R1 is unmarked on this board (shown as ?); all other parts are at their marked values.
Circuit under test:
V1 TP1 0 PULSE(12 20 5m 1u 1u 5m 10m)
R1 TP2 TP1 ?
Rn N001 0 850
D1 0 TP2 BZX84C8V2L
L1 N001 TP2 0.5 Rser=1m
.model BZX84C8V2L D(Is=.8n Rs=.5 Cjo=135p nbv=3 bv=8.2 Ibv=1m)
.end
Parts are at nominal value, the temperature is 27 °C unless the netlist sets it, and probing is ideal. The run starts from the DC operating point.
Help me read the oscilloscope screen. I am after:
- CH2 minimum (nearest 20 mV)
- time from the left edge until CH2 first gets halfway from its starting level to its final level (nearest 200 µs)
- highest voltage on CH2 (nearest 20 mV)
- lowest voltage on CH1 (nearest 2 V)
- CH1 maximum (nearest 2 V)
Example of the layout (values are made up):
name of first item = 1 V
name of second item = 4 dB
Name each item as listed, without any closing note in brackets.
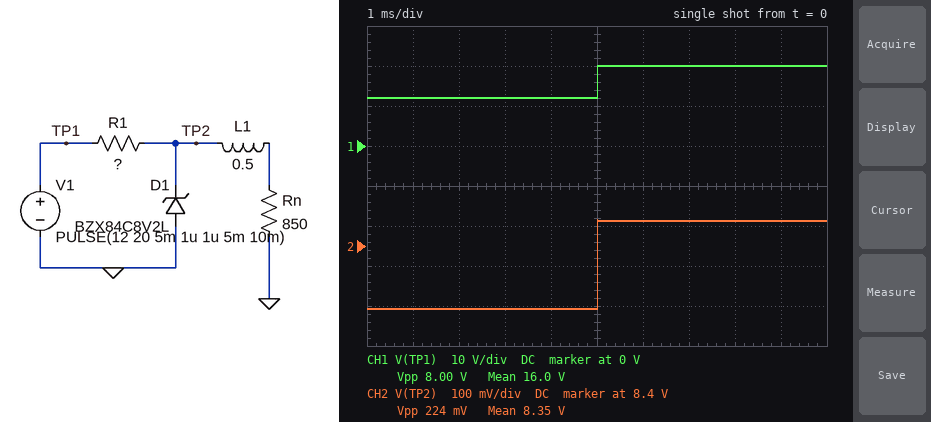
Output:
CH2 minimum = 8.24 V
time from the left edge until CH2 first gets halfway from its starting level to its final level = 5.0 ms
highest voltage on CH2 = 8.46 V
lowest voltage on CH1 = 12 V
CH1 maximum = 20 V
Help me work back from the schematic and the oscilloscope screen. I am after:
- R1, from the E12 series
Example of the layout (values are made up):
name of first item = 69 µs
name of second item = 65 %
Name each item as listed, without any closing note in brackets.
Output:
R1, from the E12 series = 330 Ω
